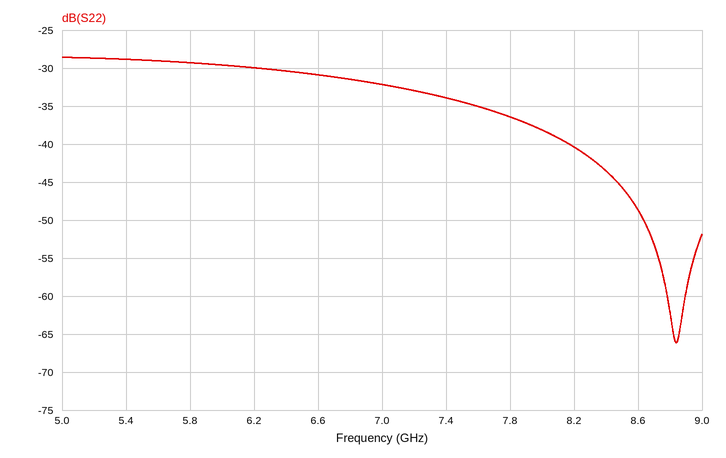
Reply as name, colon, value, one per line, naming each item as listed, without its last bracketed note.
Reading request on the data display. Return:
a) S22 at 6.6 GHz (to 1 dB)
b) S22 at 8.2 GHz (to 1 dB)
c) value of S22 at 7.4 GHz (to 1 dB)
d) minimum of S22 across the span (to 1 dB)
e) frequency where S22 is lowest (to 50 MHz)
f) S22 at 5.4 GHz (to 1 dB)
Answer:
S22 at 6.6 GHz: -31 dB
S22 at 8.2 GHz: -40 dB
value of S22 at 7.4 GHz: -34 dB
minimum of S22 across the span: -66 dB
frequency where S22 is lowest: 8.85 GHz
S22 at 5.4 GHz: -29 dB
